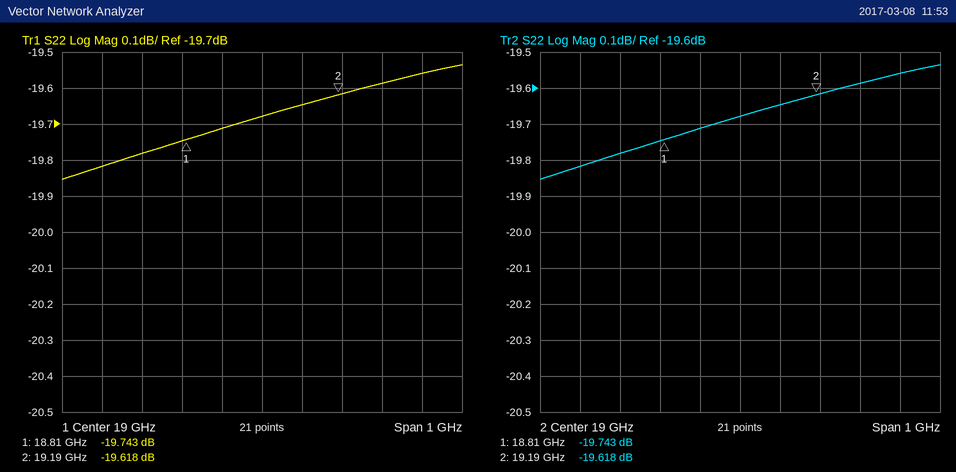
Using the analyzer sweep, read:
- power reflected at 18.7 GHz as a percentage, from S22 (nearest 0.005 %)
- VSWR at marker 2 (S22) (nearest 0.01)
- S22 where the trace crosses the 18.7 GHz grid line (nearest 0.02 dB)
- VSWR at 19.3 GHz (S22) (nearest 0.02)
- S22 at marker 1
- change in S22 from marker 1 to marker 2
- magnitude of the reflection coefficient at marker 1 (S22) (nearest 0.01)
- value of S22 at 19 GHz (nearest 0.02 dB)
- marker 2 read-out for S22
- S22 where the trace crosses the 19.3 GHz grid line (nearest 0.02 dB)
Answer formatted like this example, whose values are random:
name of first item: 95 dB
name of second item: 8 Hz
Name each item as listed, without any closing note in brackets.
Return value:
power reflected at 18.7 GHz as a percentage, from S22: 1.050 %
VSWR at marker 2 (S22): 1.23
S22 where the trace crosses the 18.7 GHz grid line: -19.78 dB
VSWR at 19.3 GHz (S22): 1.24
S22 at marker 1: -19.743 dB
change in S22 from marker 1 to marker 2: 0.125 dB
magnitude of the reflection coefficient at marker 1 (S22): 0.10
value of S22 at 19 GHz: -19.68 dB
marker 2 read-out for S22: -19.618 dB
S22 where the trace crosses the 19.3 GHz grid line: -19.58 dB
